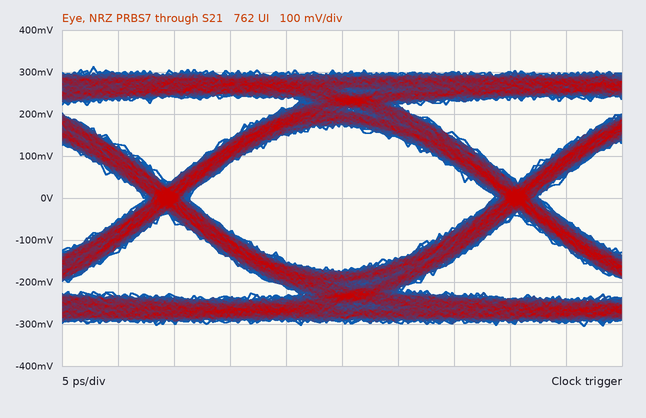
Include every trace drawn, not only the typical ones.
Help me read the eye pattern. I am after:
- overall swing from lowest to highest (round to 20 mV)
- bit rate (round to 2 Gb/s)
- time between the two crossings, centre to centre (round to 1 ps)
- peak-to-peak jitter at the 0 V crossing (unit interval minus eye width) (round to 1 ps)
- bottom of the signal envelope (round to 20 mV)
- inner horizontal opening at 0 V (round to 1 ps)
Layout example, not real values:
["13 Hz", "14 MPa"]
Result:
["620 mV", "32 Gb/s", "31 ps", "4 ps", "-300 mV", "27 ps"]
